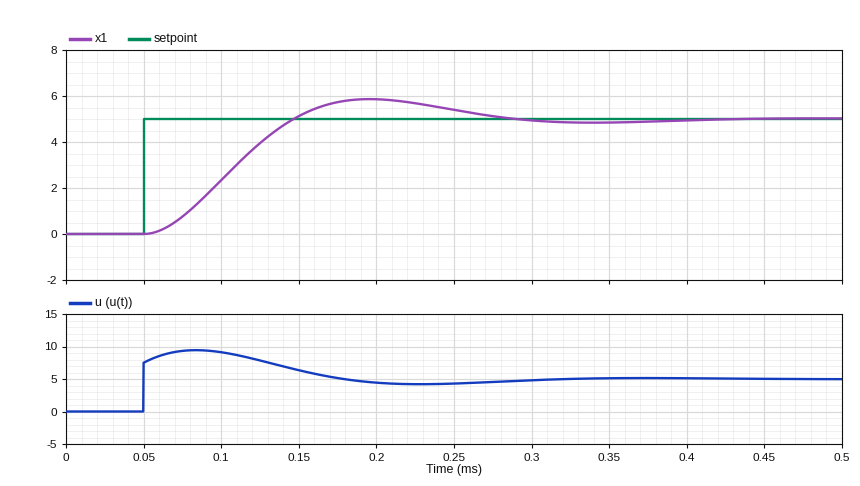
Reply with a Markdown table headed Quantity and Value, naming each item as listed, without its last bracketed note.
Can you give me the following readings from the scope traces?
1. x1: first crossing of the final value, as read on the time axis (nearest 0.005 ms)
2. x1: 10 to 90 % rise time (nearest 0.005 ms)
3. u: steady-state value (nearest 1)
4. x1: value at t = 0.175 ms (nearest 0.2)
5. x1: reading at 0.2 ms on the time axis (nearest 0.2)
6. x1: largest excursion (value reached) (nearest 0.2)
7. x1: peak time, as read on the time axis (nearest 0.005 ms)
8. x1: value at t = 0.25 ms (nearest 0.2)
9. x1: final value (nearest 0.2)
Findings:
| Quantity | Value |
|---|---|
| x1: first crossing of the final value, as read on the time axis | 0.145 ms |
| x1: 10 to 90 % rise time | 0.065 ms |
| u: steady-state value | 5 |
| x1: value at t = 0.175 ms | 5.8 |
| x1: reading at 0.2 ms on the time axis | 5.8 |
| x1: largest excursion (value reached) | 5.8 |
| x1: peak time, as read on the time axis | 0.195 ms |
| x1: value at t = 0.25 ms | 5.4 |
| x1: final value | 5.0 |
